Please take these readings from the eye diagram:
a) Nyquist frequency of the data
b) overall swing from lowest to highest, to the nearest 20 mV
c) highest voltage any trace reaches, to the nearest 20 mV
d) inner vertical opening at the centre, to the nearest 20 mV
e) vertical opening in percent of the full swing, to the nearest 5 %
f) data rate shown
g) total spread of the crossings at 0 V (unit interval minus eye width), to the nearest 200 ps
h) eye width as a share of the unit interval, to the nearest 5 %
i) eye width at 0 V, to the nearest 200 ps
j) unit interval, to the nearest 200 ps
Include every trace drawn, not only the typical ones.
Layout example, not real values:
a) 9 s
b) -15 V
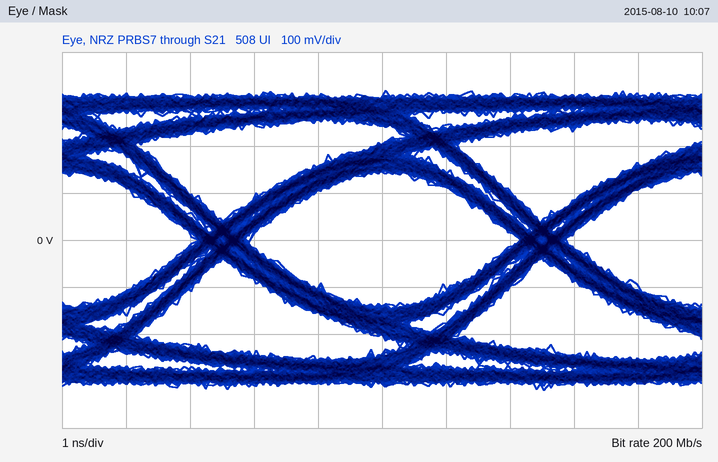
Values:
a) 100 MHz
b) 640 mV
c) 320 mV
d) 280 mV
e) 45 %
f) 200 Mb/s
g) 800 ps
h) 85 %
i) 4.2 ns
j) 5.0 ns
